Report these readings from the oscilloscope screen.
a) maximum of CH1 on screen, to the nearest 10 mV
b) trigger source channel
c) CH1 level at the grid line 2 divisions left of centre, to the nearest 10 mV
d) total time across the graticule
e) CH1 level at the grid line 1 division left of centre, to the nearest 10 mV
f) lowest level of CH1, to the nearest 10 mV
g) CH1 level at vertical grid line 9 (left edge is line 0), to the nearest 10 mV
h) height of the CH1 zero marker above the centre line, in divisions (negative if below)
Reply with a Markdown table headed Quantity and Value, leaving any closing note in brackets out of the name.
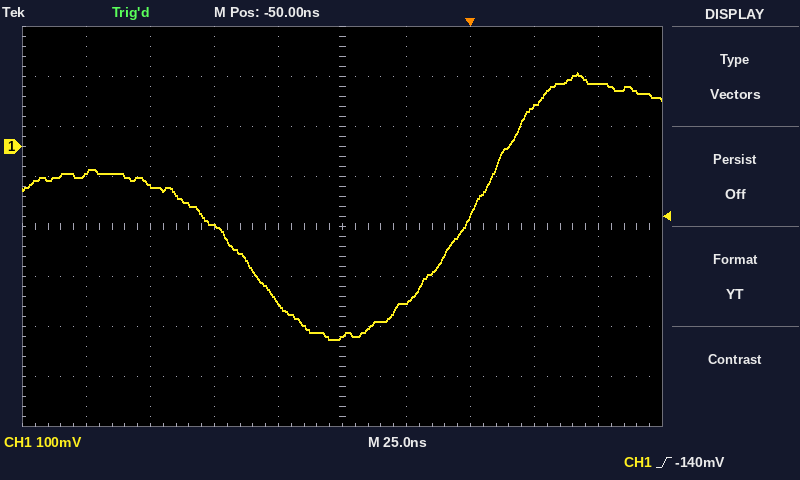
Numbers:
| Quantity | Value |
|---|---|
| maximum of CH1 on screen, to the nearest 10 mV | 150 mV |
| trigger source channel | CH1 |
| CH1 level at the grid line 2 divisions left of centre, to the nearest 10 mV | -160 mV |
| total time across the graticule | 250 ns |
| CH1 level at the grid line 1 division left of centre, to the nearest 10 mV | -310 mV |
| lowest level of CH1, to the nearest 10 mV | -390 mV |
| CH1 level at vertical grid line 9 (left edge is line 0), to the nearest 10 mV | 130 mV |
| height of the CH1 zero marker above the centre line, in divisions | +1.6 div |
